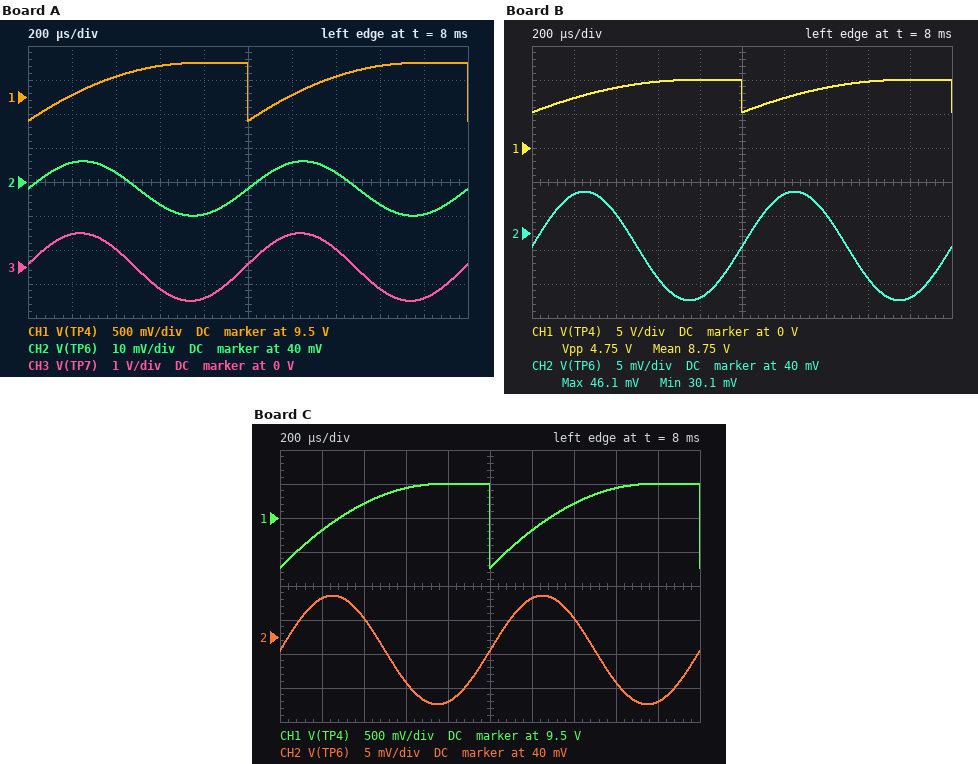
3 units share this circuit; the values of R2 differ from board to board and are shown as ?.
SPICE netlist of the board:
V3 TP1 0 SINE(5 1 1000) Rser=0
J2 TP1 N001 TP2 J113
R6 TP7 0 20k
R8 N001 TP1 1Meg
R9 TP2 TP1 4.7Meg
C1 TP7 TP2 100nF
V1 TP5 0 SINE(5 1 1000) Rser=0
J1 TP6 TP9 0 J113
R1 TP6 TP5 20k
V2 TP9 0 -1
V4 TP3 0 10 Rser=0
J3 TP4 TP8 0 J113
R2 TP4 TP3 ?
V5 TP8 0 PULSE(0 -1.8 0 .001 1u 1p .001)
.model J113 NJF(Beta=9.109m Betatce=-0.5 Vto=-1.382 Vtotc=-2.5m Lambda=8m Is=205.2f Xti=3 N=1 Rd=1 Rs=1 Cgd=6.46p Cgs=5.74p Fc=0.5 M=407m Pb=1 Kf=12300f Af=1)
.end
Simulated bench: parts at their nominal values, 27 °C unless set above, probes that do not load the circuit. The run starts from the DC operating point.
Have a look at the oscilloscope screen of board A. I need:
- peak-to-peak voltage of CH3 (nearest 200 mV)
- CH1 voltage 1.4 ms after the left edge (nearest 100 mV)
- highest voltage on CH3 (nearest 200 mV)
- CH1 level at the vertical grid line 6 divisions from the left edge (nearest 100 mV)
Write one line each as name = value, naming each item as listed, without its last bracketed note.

peak-to-peak voltage of CH3 = 2.0 V
CH1 voltage 1.4 ms after the left edge = 9.8 V
highest voltage on CH3 = 1.0 V
CH1 level at the vertical grid line 6 divisions from the left edge = 9.5 V
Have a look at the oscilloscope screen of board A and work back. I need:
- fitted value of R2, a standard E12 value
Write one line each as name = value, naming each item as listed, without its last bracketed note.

fitted value of R2, a standard E12 value = 47 Ω
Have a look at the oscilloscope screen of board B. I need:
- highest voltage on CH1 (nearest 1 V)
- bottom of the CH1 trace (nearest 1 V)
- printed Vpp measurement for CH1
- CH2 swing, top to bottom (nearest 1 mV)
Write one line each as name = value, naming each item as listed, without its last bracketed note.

highest voltage on CH1 = 10 V
bottom of the CH1 trace = 5 V
printed Vpp measurement for CH1 = 4.75 V
CH2 swing, top to bottom = 16 mV
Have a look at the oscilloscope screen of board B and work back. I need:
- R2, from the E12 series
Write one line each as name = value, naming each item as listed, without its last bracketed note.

R2, from the E12 series = 270 Ω
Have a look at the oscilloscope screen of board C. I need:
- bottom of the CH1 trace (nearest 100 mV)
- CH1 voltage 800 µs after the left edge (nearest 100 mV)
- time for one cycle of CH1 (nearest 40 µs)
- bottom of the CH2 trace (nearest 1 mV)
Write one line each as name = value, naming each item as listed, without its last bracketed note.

bottom of the CH1 trace = 8.8 V
CH1 voltage 800 µs after the left edge = 10.0 V
time for one cycle of CH1 = 1.00 ms
bottom of the CH2 trace = 30 mV
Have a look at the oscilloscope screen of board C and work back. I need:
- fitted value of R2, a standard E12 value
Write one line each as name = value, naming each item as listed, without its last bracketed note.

fitted value of R2, a standard E12 value = 68 Ω
